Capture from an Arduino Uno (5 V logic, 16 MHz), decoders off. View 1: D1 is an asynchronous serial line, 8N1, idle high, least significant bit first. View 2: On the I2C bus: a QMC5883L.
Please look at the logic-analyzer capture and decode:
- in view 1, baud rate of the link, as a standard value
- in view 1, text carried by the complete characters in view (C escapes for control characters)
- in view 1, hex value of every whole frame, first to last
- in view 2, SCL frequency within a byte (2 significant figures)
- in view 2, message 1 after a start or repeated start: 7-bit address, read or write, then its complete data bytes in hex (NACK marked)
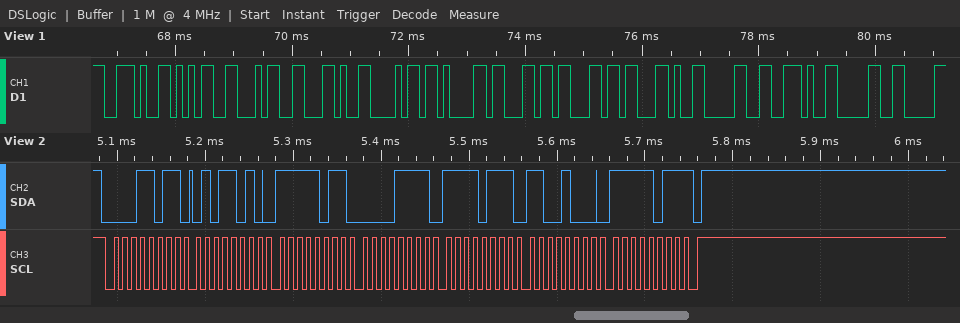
9600 baud
".54,hall,0.0"
2E 35 34 2C 68 61 6C 6C 2C 30 2E 30
100 kHz
0x0D read: 5A FB 0F F7 C8 FB NACK
